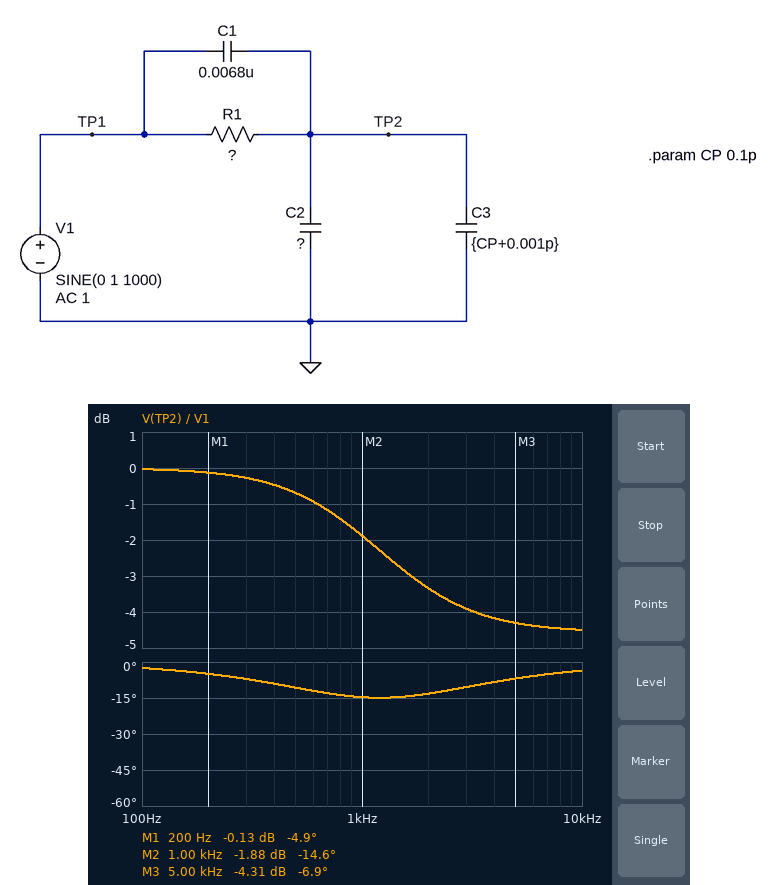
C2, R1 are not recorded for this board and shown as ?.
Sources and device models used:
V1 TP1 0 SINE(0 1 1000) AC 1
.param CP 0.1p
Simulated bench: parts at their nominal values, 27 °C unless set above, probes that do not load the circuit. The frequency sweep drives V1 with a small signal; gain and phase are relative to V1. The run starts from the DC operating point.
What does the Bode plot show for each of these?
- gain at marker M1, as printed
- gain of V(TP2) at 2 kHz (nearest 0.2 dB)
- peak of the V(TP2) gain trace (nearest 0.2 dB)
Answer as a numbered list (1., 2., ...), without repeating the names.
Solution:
1. -0.13 dB
2. -3.4 dB
3. 0 dB
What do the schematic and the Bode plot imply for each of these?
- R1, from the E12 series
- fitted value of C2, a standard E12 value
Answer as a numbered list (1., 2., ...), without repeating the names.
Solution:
1. 15 kΩ
2. 4.7 nF
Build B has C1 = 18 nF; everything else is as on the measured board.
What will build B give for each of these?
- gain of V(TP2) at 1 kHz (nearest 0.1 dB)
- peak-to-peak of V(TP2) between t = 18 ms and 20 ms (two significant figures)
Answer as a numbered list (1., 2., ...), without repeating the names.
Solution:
1. -1.6 dB
2. 1.7 V
